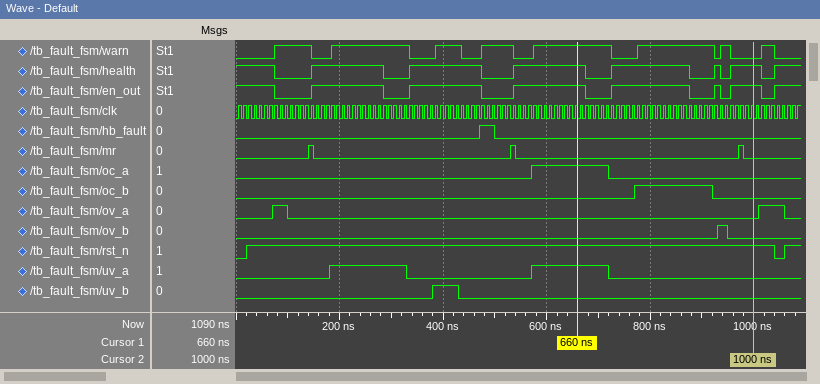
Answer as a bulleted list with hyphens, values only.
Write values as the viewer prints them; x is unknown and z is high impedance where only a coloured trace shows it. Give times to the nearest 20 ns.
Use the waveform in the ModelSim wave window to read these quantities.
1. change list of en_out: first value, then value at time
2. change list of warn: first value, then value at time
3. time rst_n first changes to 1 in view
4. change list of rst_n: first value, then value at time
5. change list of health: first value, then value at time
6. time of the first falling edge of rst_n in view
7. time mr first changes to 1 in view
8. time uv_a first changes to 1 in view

- 1, 0 at 80 ns, 1 at 140 ns, 0 at 280 ns, 1 at 340 ns, 0 at 480 ns, 1 at 540 ns, 0 at 680 ns, 1 at 720 ns, 0 at 880 ns, 1 at 920 ns, 0 at 940 ns, 1 at 960 ns, 0 at 1020 ns, 1 at 1040 ns
- 0, 1 at 80 ns, 0 at 140 ns, 1 at 180 ns, 0 at 340 ns, 1 at 380 ns, 0 at 440 ns, 1 at 480 ns, 0 at 540 ns, 1 at 580 ns, 0 at 720 ns, 1 at 780 ns, 0 at 920 ns, 1 at 940 ns, 0 at 960 ns, 1 at 1020 ns, 0 at 1040 ns
- 20 ns
- 0, 1 at 20 ns, 0 at 1040 ns, 1 at 1060 ns
- 1, 0 at 80 ns, 1 at 140 ns, 0 at 280 ns, 1 at 340 ns, 0 at 480 ns, 1 at 540 ns, 0 at 680 ns, 1 at 720 ns, 0 at 880 ns, 1 at 920 ns, 0 at 940 ns, 1 at 960 ns, 0 at 1020 ns, 1 at 1040 ns
- 1040 ns
- 140 ns
- 180 ns
